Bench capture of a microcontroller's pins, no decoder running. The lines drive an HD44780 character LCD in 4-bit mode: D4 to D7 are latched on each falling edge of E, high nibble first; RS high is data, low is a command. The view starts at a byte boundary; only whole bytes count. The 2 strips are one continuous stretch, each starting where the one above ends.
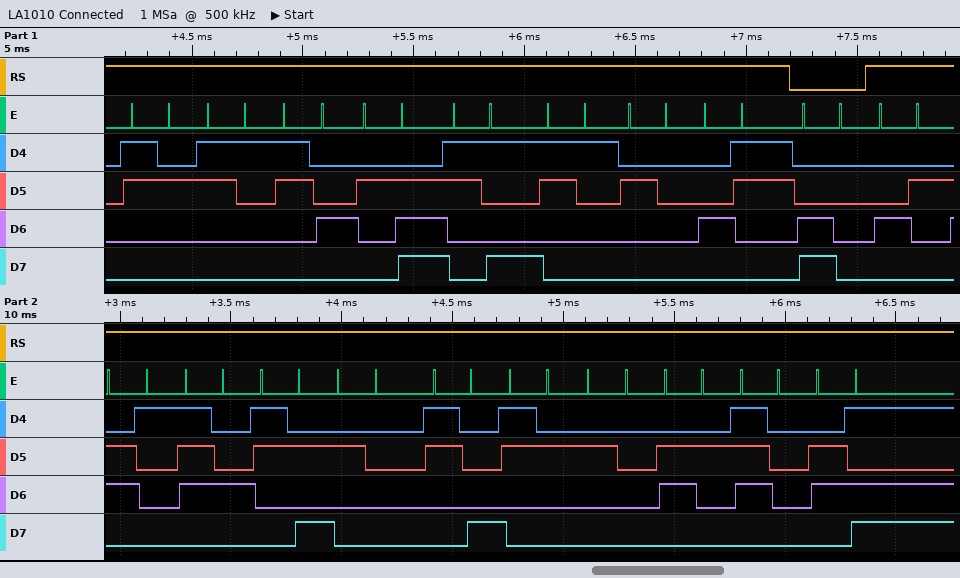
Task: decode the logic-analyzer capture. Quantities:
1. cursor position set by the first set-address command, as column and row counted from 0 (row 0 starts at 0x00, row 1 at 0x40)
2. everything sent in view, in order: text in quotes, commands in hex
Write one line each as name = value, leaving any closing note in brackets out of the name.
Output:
cursor position set by the first set-address command, as column and row counted from 0 = column 0, row 1
everything sent in view, in order: text in quotes, commands in hex = "214.91 C" 0xC0 "Bat: 82 bpm"
